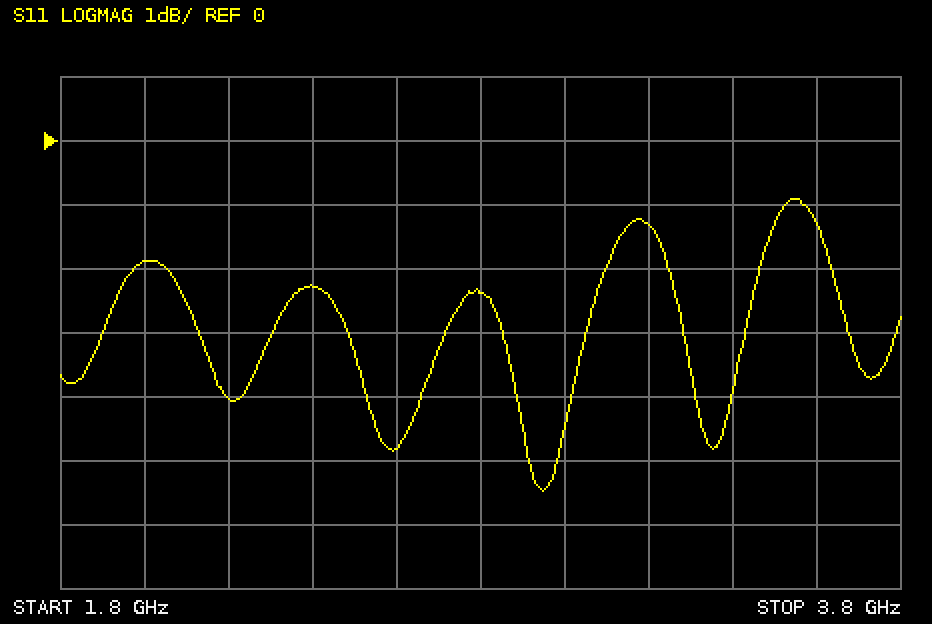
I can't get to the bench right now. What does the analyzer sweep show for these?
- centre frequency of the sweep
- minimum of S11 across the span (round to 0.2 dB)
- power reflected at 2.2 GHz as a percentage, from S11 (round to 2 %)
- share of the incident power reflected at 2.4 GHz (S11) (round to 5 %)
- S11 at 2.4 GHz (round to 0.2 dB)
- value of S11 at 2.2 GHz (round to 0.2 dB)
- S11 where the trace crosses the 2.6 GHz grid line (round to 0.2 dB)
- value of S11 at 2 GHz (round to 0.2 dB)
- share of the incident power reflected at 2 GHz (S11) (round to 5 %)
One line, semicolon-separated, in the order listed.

2.8 GHz; -5.4 dB; 40 %; 60 %; -2.2 dB; -4.0 dB; -4.8 dB; -1.8 dB; 65 %
